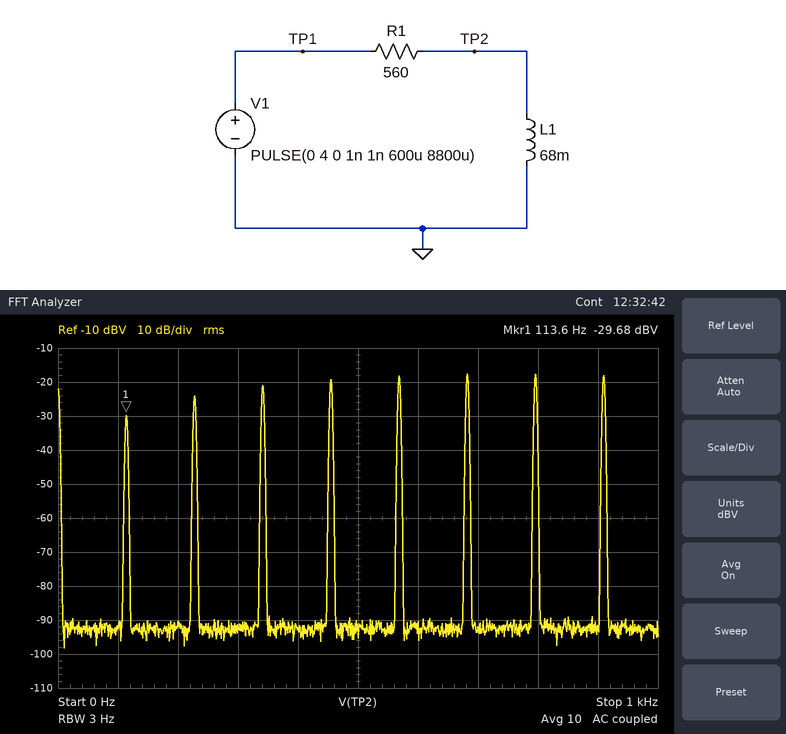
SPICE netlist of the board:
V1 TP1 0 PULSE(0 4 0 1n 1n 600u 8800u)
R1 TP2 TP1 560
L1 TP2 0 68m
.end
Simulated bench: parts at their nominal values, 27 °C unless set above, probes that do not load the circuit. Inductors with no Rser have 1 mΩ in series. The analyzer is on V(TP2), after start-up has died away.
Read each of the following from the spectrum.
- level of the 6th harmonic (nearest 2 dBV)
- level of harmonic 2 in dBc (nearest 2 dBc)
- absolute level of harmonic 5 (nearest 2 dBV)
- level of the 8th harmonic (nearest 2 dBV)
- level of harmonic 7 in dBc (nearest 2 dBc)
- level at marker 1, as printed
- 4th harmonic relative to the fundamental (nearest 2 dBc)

-18 dBV
6 dBc
-18 dBV
-18 dBV
12 dBc
-29.68 dBV
10 dBc
